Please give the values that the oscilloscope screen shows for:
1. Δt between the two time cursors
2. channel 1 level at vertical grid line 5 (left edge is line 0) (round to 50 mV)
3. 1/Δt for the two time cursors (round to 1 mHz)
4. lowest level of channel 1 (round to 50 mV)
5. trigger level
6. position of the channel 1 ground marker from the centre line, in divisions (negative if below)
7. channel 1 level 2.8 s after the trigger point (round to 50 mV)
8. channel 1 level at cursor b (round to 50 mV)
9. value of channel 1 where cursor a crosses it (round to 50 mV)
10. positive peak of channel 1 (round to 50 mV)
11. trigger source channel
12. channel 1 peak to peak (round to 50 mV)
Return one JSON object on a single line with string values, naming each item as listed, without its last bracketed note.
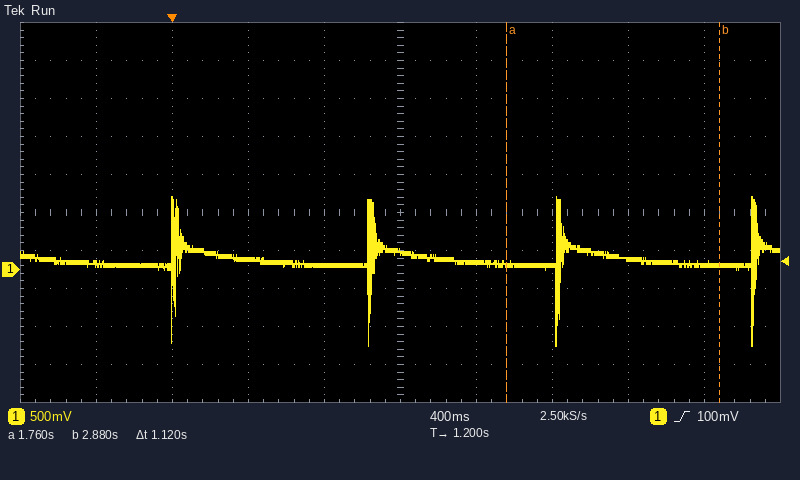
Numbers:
{"Δt between the two time cursors": "1.12 s", "channel 1 level at vertical grid line 5 (left edge is line 0)": "250 mV", "1/Δt for the two time cursors": "893 mHz", "lowest level of channel 1": "-1.00 V", "trigger level": "100 mV", "position of the channel 1 ground marker from the centre line, in divisions": "-1.5 div", "channel 1 level 2.8 s after the trigger point": "50 mV", "channel 1 level at cursor b": "50 mV", "value of channel 1 where cursor a crosses it": "100 mV", "positive peak of channel 1": "950 mV", "trigger source channel": "channel 1", "channel 1 peak to peak": "1.95 V"}
